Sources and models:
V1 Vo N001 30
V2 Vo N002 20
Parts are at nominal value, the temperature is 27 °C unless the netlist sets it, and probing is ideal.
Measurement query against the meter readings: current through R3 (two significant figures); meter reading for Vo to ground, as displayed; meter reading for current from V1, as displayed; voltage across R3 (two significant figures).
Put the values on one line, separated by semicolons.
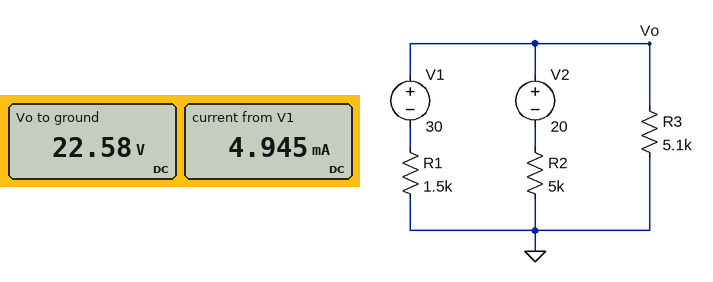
4.4 mA; 22.58 V; 4.945 mA; 23 V
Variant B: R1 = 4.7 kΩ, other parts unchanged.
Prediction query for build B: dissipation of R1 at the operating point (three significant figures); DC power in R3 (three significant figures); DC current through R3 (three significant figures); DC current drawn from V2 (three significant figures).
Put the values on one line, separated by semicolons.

35.7 mW; 57.0 mW; 3.34 mA; 589 µA
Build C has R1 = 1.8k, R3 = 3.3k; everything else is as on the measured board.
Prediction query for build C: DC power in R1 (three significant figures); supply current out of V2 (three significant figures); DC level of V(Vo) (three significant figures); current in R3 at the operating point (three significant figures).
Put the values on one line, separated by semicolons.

61.0 mW; 95.4 µA; 19.5 V; 5.92 mA
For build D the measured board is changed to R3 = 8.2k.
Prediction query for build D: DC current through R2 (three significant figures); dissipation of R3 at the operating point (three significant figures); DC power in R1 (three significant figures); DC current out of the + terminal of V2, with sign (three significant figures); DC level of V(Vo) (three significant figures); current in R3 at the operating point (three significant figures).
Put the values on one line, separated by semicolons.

855 µA; 71.9 mW; 21.8 mW; -855 µA; 24.3 V; 2.96 mA
